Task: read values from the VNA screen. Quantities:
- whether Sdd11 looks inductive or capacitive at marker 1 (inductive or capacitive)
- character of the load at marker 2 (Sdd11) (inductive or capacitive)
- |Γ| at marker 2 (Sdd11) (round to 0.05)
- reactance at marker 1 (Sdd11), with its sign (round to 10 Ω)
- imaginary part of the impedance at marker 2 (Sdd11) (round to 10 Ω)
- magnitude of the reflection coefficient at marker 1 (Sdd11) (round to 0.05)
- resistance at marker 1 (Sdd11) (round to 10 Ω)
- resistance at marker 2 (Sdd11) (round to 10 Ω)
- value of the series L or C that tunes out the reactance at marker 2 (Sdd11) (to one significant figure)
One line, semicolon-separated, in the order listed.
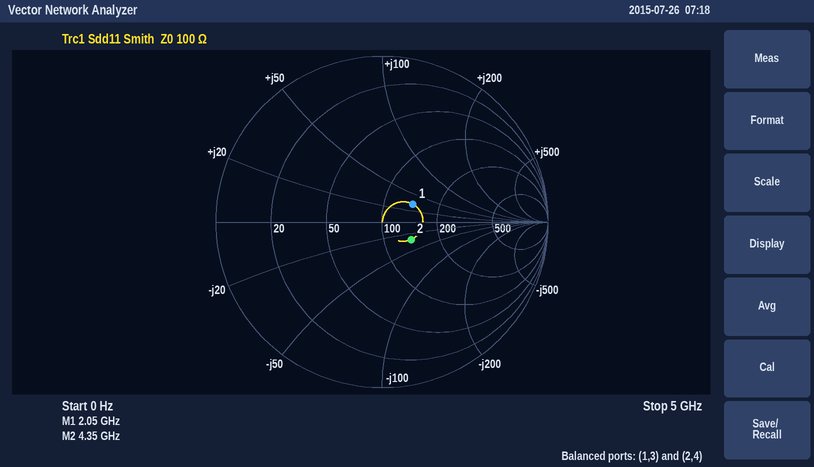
inductive; capacitive; 0.20; +30 Ω; -30 Ω; 0.20; 140 Ω; 140 Ω; 1 nH
